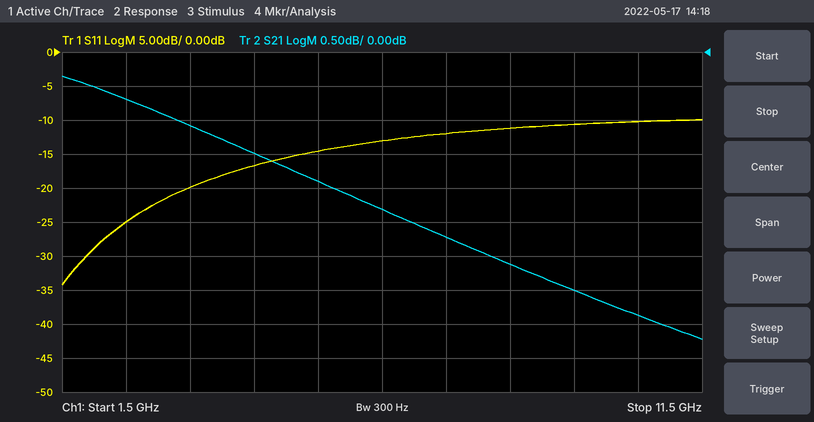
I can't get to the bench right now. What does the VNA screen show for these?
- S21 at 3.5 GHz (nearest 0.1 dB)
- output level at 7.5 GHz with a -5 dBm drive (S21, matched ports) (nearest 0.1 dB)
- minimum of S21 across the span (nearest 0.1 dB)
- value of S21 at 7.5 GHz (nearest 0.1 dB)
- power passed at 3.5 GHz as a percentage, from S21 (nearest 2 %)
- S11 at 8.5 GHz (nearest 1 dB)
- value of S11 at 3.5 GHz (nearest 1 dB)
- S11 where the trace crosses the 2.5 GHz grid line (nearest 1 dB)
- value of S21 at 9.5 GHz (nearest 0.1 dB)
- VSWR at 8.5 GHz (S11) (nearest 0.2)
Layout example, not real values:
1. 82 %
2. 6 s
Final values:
1. -1.1 dB
2. -7.7 dBm
3. -4.2 dB
4. -2.7 dB
5. 78 %
6. -11 dB
7. -20 dB
8. -25 dB
9. -3.5 dB
10. 1.8
